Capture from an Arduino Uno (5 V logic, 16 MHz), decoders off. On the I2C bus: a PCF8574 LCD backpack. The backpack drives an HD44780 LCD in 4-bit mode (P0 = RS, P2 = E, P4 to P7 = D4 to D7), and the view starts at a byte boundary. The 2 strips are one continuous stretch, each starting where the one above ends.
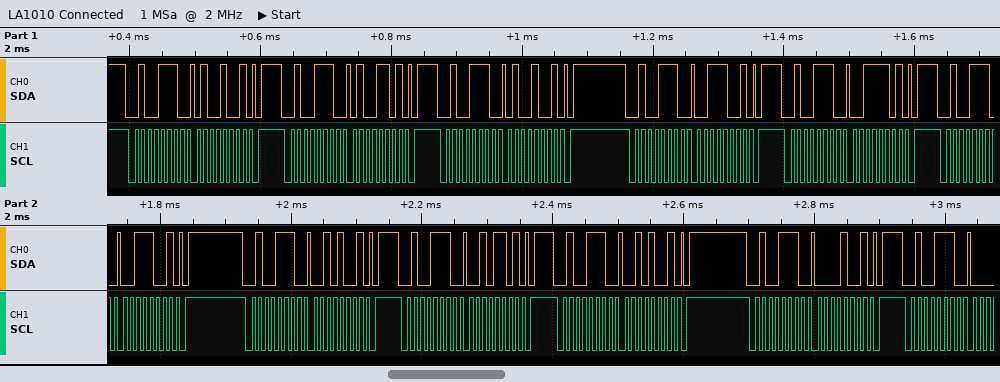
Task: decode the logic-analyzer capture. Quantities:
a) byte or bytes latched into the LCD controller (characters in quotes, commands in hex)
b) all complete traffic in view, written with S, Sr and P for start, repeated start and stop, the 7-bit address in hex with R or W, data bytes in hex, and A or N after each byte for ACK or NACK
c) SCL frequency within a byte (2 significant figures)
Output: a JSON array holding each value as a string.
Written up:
["'C'", "S 27W A 49 A P S 27W A 4D A P S 27W A 49 A P S 27W A 39 A P S 27W A 3D A P S 27W A 39 A P S 27W A 29 A P S 27W A 2D A P S 27W A 29 A P S 27W A 09 A P S 27W A", "100 kHz"]
